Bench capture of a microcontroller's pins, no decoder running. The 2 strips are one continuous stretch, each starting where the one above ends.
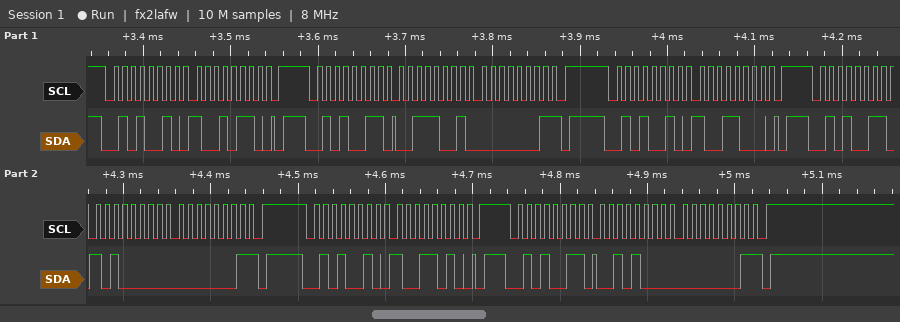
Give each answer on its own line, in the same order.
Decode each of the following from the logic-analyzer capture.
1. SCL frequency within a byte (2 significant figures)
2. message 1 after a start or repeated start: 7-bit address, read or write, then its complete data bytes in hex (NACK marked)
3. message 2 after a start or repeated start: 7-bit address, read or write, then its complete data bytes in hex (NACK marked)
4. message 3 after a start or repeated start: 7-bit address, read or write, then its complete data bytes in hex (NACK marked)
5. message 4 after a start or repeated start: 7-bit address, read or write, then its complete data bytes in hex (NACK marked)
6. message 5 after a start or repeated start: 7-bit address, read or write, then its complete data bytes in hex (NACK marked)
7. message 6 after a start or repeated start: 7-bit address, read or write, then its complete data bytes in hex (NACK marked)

100 kHz
0x29 write: 96
0x29 read: 39 01 NACK
0x29 write: 98
0x29 read: A0 01 NACK
0x29 write: 9A
0x29 read: 28 01 NACK
